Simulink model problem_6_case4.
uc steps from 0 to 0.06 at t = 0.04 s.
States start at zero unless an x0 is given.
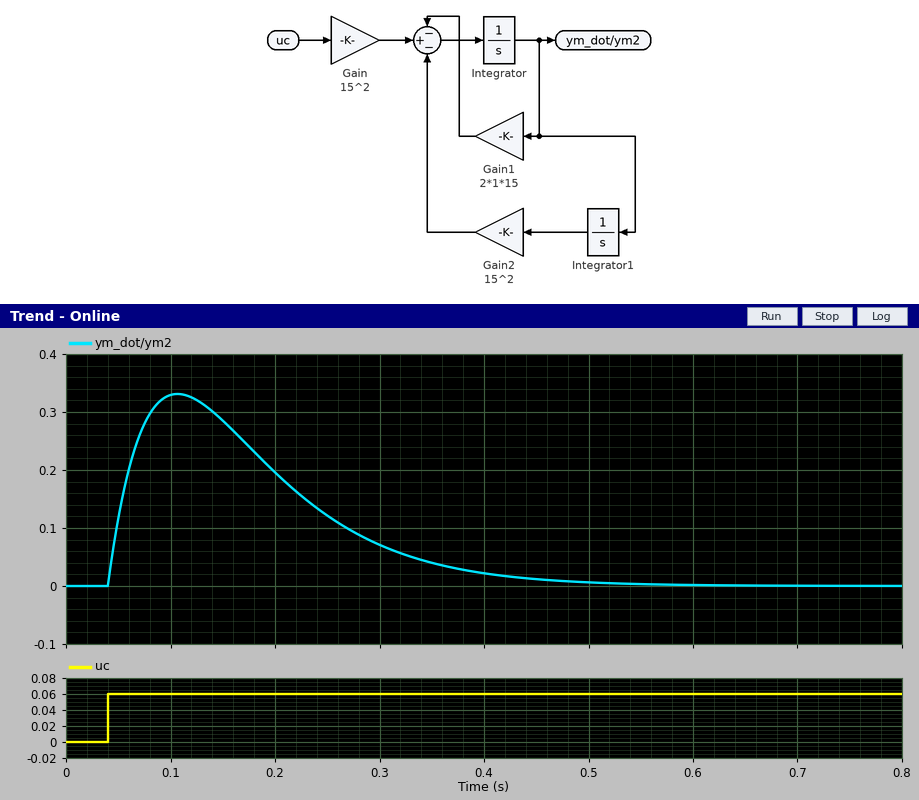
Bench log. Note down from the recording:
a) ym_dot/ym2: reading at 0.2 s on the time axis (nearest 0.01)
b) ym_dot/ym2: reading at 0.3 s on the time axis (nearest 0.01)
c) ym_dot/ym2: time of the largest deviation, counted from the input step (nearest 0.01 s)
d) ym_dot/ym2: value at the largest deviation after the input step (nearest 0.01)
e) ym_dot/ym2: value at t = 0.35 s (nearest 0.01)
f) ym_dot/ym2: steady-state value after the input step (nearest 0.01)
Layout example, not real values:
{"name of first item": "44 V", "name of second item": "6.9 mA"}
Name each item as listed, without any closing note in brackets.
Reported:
{"ym_dot/ym2: reading at 0.2 s on the time axis": "0.20", "ym_dot/ym2: reading at 0.3 s on the time axis": "0.07", "ym_dot/ym2: time of the largest deviation, counted from the input step": "0.07 s", "ym_dot/ym2: value at the largest deviation after the input step": "0.33", "ym_dot/ym2: value at t = 0.35 s": "0.04", "ym_dot/ym2: steady-state value after the input step": "0.00"}
